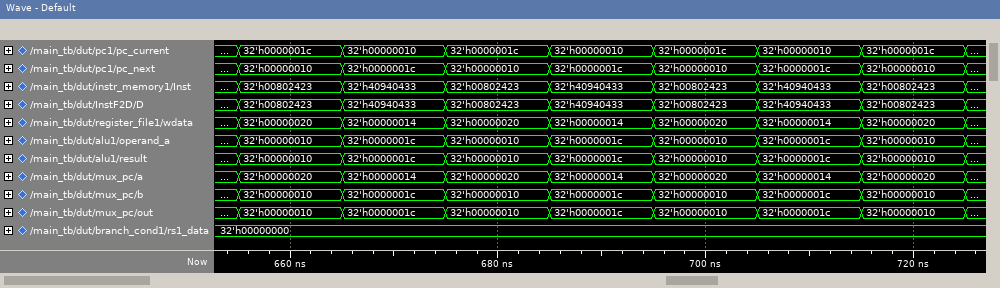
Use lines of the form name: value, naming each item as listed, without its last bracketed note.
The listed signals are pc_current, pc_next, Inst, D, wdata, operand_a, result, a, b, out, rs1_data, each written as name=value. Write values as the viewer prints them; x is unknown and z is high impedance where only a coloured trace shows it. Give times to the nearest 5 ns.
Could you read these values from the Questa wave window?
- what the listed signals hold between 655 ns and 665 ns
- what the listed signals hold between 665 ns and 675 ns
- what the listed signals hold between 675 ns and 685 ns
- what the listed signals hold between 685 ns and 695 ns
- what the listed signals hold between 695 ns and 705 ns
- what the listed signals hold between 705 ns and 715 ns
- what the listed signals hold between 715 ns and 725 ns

what the listed signals hold between 655 ns and 665 ns: pc_current=32'h0000001c, pc_next=32'h00000010, Inst=32'h00802423, D=32'h00802423, wdata=32'h00000020, operand_a=32'h00000010, result=32'h00000010, a=32'h00000020, b=32'h00000010, out=32'h00000010, rs1_data=32'h00000000
what the listed signals hold between 665 ns and 675 ns: pc_current=32'h00000010, pc_next=32'h0000001c, Inst=32'h40940433, D=32'h40940433, wdata=32'h00000014, operand_a=32'h0000001c, result=32'h0000001c, a=32'h00000014, b=32'h0000001c, out=32'h0000001c, rs1_data=32'h00000000
what the listed signals hold between 675 ns and 685 ns: pc_current=32'h0000001c, pc_next=32'h00000010, Inst=32'h00802423, D=32'h00802423, wdata=32'h00000020, operand_a=32'h00000010, result=32'h00000010, a=32'h00000020, b=32'h00000010, out=32'h00000010, rs1_data=32'h00000000
what the listed signals hold between 685 ns and 695 ns: pc_current=32'h00000010, pc_next=32'h0000001c, Inst=32'h40940433, D=32'h40940433, wdata=32'h00000014, operand_a=32'h0000001c, result=32'h0000001c, a=32'h00000014, b=32'h0000001c, out=32'h0000001c, rs1_data=32'h00000000
what the listed signals hold between 695 ns and 705 ns: pc_current=32'h0000001c, pc_next=32'h00000010, Inst=32'h00802423, D=32'h00802423, wdata=32'h00000020, operand_a=32'h00000010, result=32'h00000010, a=32'h00000020, b=32'h00000010, out=32'h00000010, rs1_data=32'h00000000
what the listed signals hold between 705 ns and 715 ns: pc_current=32'h00000010, pc_next=32'h0000001c, Inst=32'h40940433, D=32'h40940433, wdata=32'h00000014, operand_a=32'h0000001c, result=32'h0000001c, a=32'h00000014, b=32'h0000001c, out=32'h0000001c, rs1_data=32'h00000000
what the listed signals hold between 715 ns and 725 ns: pc_current=32'h0000001c, pc_next=32'h00000010, Inst=32'h00802423, D=32'h00802423, wdata=32'h00000020, operand_a=32'h00000010, result=32'h00000010, a=32'h00000020, b=32'h00000010, out=32'h00000010, rs1_data=32'h00000000
